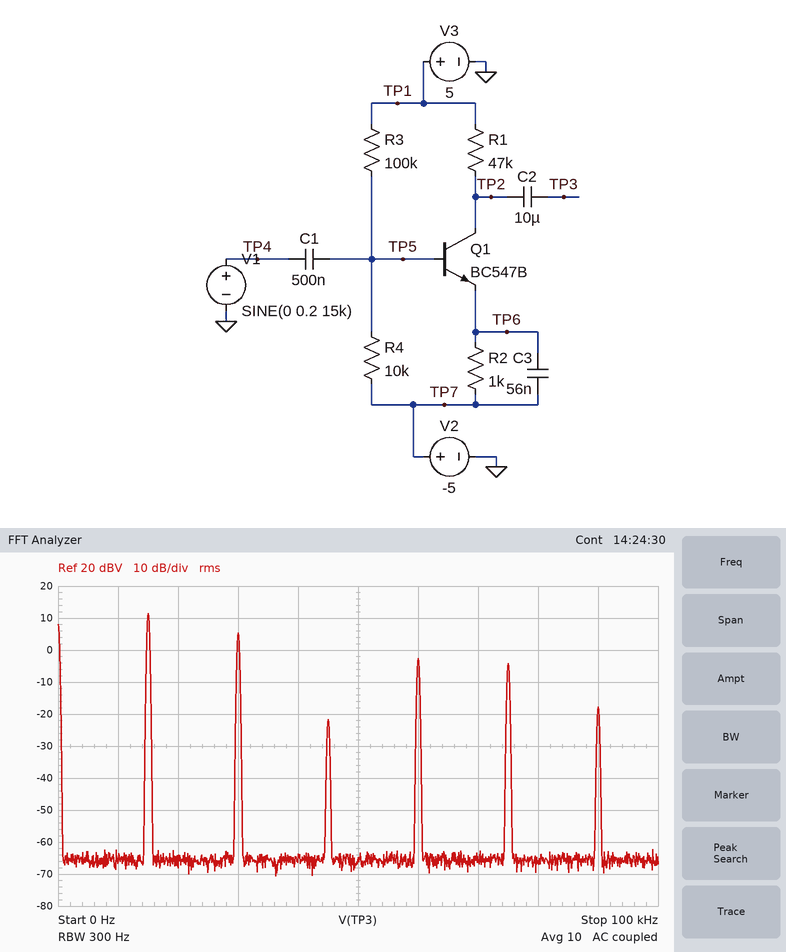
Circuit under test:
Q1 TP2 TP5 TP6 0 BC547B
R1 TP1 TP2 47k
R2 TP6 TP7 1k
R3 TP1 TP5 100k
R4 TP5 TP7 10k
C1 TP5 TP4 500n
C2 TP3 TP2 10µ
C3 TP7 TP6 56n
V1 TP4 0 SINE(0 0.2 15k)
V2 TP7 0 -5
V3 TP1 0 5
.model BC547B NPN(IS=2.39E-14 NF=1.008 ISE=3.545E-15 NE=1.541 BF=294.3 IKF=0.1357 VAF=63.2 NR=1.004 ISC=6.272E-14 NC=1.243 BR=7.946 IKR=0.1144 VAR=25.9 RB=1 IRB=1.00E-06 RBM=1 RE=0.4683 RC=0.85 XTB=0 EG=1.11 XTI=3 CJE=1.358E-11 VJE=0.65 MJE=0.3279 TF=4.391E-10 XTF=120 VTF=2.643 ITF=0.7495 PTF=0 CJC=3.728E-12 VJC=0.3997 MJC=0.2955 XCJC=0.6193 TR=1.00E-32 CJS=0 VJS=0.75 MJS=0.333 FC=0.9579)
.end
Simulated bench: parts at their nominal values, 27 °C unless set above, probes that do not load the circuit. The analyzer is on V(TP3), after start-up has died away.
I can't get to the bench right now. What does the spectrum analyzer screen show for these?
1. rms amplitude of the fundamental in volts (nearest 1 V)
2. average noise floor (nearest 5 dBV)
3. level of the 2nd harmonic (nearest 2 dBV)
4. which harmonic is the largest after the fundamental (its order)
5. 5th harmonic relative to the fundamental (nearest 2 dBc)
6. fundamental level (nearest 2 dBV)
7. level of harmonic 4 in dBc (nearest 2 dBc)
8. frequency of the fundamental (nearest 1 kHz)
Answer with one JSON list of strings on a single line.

["4 V", "-65 dBV", "6 dBV", "2", "-16 dBc", "12 dBV", "-14 dBc", "15 kHz"]
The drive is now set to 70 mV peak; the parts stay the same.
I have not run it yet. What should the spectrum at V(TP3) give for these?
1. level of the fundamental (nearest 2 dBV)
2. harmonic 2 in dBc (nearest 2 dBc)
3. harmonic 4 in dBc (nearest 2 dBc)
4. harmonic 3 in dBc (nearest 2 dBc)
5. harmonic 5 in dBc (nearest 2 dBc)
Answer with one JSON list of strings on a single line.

["12 dBV", "-26 dBc", "-32 dBc", "-14 dBc", "-22 dBc"]
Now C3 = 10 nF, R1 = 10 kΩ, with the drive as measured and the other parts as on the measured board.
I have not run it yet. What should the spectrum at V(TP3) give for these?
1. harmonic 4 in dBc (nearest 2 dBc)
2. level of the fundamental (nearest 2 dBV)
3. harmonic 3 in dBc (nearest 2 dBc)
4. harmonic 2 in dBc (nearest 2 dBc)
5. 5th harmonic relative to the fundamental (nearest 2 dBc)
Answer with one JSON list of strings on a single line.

["-44 dBc", "4 dBV", "-36 dBc", "-26 dBc", "-52 dBc"]
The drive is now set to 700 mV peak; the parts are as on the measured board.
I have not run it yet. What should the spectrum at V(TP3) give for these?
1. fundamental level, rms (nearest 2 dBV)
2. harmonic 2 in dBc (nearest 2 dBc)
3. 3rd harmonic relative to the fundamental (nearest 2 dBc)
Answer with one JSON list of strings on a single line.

["8 dBV", "-2 dBc", "-6 dBc"]
